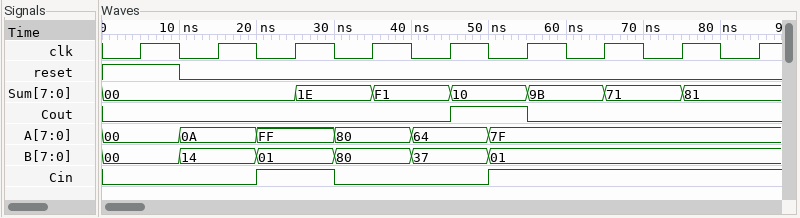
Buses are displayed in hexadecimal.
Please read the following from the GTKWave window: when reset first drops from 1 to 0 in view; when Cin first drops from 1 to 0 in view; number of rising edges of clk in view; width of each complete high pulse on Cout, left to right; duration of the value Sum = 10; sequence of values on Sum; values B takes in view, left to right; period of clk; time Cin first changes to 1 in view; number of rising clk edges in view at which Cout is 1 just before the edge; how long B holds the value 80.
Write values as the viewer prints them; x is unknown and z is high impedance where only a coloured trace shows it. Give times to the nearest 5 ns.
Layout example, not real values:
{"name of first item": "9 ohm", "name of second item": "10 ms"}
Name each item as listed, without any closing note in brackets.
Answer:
{"when reset first drops from 1 to 0 in view": "10 ns", "when Cin first drops from 1 to 0 in view": "30 ns", "number of rising edges of clk in view": "9", "width of each complete high pulse on Cout, left to right": "10 ns", "duration of the value Sum = 10": "10 ns", "sequence of values on Sum": "00, 1E, F1, 10, 9B, 71, 81", "values B takes in view, left to right": "00, 14, 01, 80, 37, 01", "period of clk": "10 ns", "time Cin first changes to 1 in view": "20 ns", "number of rising clk edges in view at which Cout is 1 just before the edge": "1", "how long B holds the value 80": "10 ns"}
